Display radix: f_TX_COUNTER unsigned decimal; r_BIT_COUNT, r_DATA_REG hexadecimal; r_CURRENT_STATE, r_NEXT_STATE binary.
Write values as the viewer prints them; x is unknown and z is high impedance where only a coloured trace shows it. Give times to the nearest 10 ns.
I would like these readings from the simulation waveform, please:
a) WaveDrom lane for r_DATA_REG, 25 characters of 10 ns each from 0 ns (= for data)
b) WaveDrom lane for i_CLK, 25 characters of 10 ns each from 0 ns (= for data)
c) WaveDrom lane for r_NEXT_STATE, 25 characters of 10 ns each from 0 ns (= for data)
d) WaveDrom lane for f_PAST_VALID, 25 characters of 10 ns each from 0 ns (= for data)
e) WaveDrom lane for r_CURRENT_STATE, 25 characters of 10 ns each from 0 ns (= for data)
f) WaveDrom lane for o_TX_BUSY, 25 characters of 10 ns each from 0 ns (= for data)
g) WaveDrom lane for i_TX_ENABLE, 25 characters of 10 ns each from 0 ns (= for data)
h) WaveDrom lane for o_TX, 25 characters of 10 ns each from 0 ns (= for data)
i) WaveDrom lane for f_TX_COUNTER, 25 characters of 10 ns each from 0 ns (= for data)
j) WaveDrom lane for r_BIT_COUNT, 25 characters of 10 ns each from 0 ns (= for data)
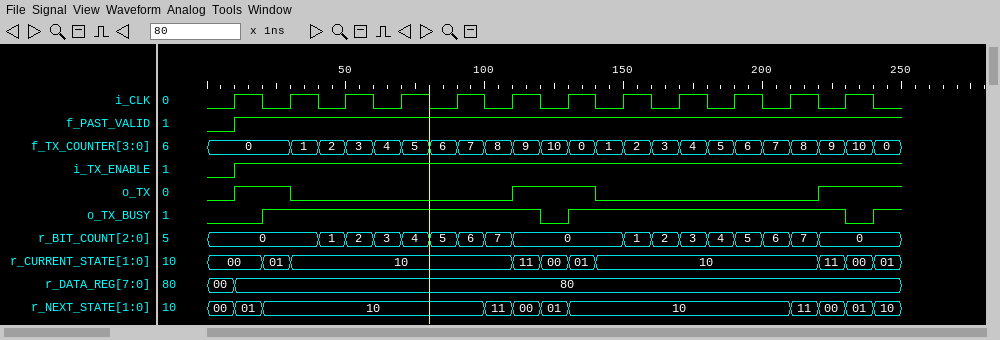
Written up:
{name: 'r_DATA_REG', wave: '==.......................', data: '00 80'}
{name: 'i_CLK', wave: '0101010101010101010101010'}
{name: 'r_NEXT_STATE', wave: '===.......====.......====', data: '00 01 10 11 00 01 10 11 00 01 10'}
{name: 'f_PAST_VALID', wave: '01.......................'}
{name: 'r_CURRENT_STATE', wave: '=.==.......====.......===', data: '00 01 10 11 00 01 10 11 00 01'}
{name: 'o_TX_BUSY', wave: '0.1.........01.........01'}
{name: 'i_TX_ENABLE', wave: '01.......................'}
{name: 'o_TX', wave: '01.0.......1..0.......1..'}
{name: 'f_TX_COUNTER', wave: '=..======================', data: '0 1 2 3 4 5 6 7 8 9 10 0 1 2 3 4 5 6 7 8 9 10 0'}
{name: 'r_BIT_COUNT', wave: '=...========...========..', data: '0 1 2 3 4 5 6 7 0 1 2 3 4 5 6 7 0'}
